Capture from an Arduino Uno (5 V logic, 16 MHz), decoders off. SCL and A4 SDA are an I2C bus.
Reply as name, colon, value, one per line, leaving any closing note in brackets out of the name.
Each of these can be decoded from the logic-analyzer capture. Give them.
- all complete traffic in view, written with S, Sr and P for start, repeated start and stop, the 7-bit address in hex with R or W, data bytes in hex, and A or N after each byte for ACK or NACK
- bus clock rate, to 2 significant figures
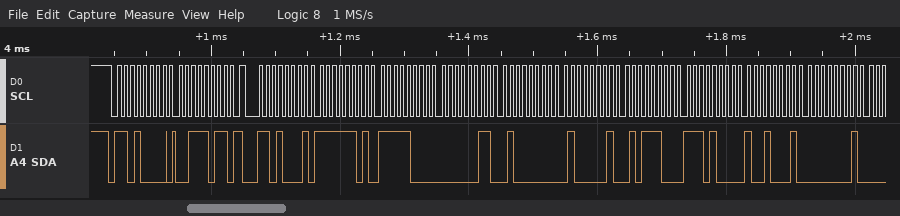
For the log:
all complete traffic in view, written with S, Sr and P for start, repeated start and stop, the 7-bit address in hex with R or W, data bytes in hex, and A or N after each byte for ACK or NACK: S 68W A 3B A Sr 68R A FD A F8 A 03 A 40 A 41 A 5C A E8 A 91 A 01 A
bus clock rate, to 2 significant figures: 100 kHz
